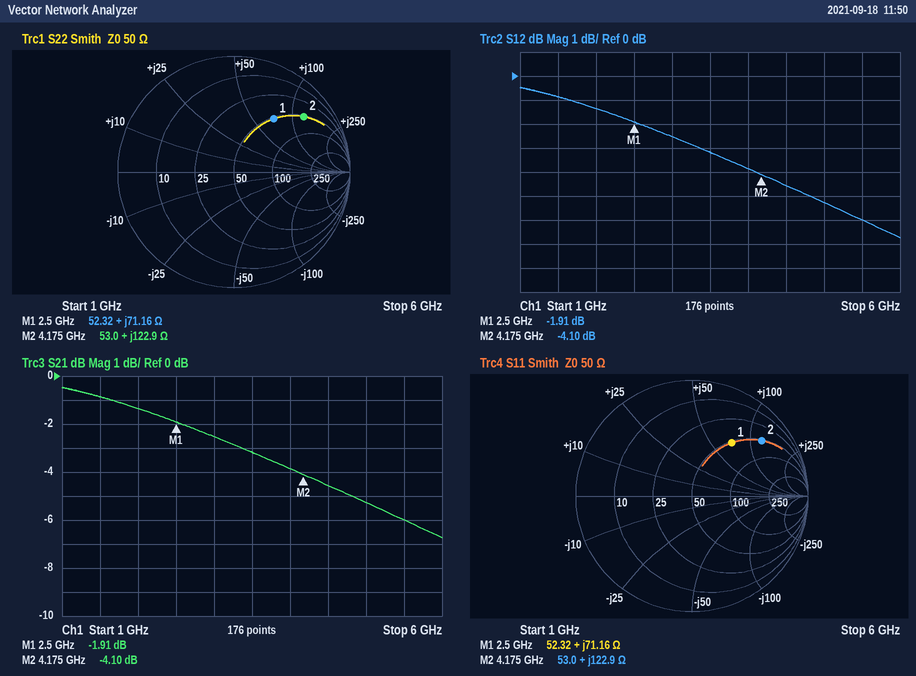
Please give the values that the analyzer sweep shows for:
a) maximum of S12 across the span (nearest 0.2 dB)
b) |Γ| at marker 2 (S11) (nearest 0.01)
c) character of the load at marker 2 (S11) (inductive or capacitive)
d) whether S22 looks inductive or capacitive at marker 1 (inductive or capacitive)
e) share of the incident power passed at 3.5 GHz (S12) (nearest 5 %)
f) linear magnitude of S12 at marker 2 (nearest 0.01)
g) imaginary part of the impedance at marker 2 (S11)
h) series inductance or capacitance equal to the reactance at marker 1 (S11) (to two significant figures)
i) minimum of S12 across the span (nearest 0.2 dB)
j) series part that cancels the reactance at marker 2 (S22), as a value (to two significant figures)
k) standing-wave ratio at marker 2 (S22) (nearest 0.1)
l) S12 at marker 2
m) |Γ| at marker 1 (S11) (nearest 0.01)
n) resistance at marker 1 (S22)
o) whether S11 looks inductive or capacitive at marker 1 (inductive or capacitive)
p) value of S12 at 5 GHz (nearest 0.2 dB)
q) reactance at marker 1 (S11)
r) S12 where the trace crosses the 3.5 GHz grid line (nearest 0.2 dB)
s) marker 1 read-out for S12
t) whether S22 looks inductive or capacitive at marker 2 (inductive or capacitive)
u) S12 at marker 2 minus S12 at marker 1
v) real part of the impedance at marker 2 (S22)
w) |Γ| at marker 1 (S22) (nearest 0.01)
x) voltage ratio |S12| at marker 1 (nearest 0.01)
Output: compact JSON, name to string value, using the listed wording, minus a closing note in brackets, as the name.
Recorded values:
{"maximum of S12 across the span": "-0.4 dB", "|Γ| at marker 2 (S11)": "0.77", "character of the load at marker 2 (S11)": "inductive", "whether S22 looks inductive or capacitive at marker 1": "inductive", "share of the incident power passed at 3.5 GHz (S12)": "50 %", "linear magnitude of S12 at marker 2": "0.62", "imaginary part of the impedance at marker 2": "+122.9 Ω", "series inductance or capacitance equal to the reactance at marker 1 (S11)": "4.5 nH", "minimum of S12 across the span": "-6.8 dB", "series part that cancels the reactance at marker 2 (S22), as a value": "310 fF", "standing-wave ratio at marker 2 (S22)": "7.6", "S12 at marker 2": "-4.10 dB", "|Γ| at marker 1 (S11)": "0.57", "resistance at marker 1": "52.32 Ω", "whether S11 looks inductive or capacitive at marker 1": "inductive", "value of S12 at 5 GHz": "-5.2 dB", "reactance at marker 1": "+71.16 Ω", "S12 where the trace crosses the 3.5 GHz grid line": "-3.2 dB", "marker 1 read-out for S12": "-1.91 dB", "whether S22 looks inductive or capacitive at marker 2": "inductive", "S12 at marker 2 minus S12 at marker 1": "-2.19 dB", "real part of the impedance at marker 2": "53.0 Ω", "|Γ| at marker 1 (S22)": "0.57", "voltage ratio |S12| at marker 1": "0.80"}
